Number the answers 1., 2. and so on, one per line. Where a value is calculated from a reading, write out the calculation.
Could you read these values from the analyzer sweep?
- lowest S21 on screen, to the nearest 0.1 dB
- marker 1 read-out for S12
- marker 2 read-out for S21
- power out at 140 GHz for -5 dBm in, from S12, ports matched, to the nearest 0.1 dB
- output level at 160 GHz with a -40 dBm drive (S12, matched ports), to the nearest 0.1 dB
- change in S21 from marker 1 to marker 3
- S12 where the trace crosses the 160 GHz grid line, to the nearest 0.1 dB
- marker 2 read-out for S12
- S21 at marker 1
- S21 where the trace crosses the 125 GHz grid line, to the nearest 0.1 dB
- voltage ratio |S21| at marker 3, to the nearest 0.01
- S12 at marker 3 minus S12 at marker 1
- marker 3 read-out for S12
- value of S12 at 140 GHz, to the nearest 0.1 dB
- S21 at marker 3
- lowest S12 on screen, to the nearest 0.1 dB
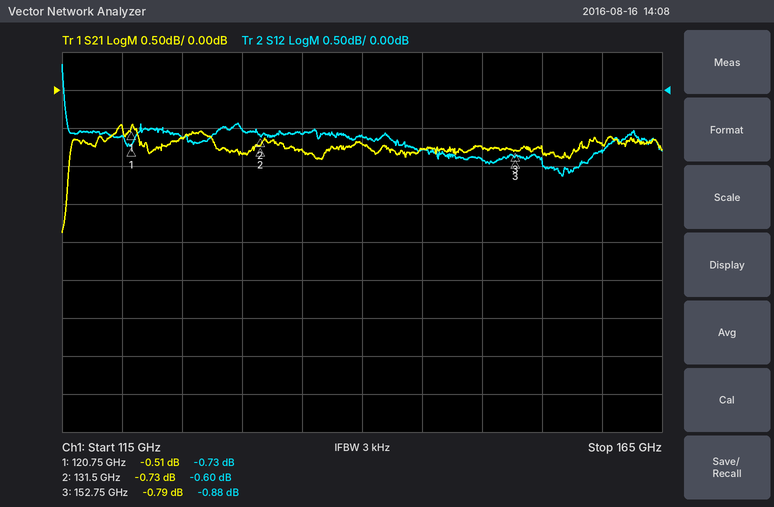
1. -1.9 dB
2. -0.73 dB
3. -0.73 dB
4. -5 dBm + (-0.6 dB) = -5.6 dBm
5. -40 dBm + (-0.8 dB) = -40.8 dBm
6. -0.79 − (-0.51) = -0.28 dB
7. -0.8 dB
8. -0.60 dB
9. -0.51 dB
10. -0.6 dB
11. 10^(-0.79/20) ≈ 0.91
12. -0.88 − (-0.73) = -0.15 dB
13. -0.88 dB
14. -0.6 dB
15. -0.79 dB
16. -1.1 dB
